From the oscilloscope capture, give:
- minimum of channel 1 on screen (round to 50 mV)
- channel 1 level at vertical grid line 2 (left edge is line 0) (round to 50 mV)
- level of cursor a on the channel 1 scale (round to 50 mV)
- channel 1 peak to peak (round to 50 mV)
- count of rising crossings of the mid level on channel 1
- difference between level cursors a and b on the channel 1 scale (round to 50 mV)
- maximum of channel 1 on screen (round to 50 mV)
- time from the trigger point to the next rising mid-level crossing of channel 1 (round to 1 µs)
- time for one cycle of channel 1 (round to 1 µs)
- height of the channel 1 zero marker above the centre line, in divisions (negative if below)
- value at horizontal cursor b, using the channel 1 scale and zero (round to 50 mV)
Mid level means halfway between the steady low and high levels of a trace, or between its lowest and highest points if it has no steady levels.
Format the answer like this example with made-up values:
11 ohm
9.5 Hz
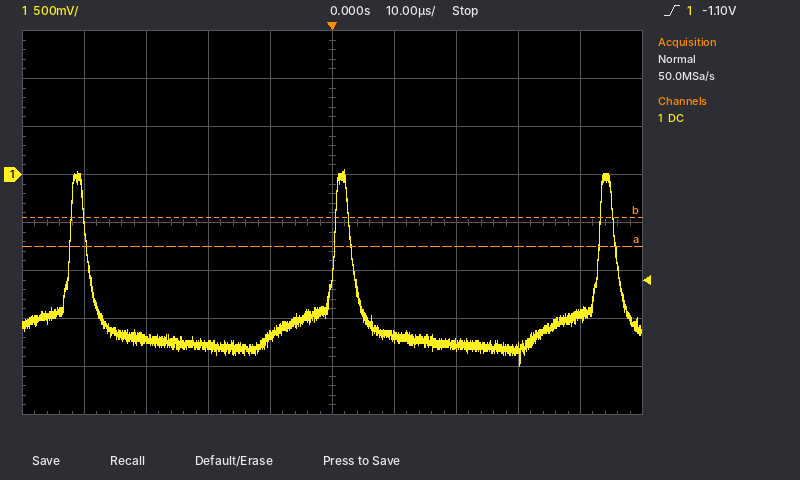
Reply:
-2.00 V
-1.70 V
-750 mV
2.05 V
3
300 mV
50 mV
43 µs
43 µs
+1.0 div
-450 mV
